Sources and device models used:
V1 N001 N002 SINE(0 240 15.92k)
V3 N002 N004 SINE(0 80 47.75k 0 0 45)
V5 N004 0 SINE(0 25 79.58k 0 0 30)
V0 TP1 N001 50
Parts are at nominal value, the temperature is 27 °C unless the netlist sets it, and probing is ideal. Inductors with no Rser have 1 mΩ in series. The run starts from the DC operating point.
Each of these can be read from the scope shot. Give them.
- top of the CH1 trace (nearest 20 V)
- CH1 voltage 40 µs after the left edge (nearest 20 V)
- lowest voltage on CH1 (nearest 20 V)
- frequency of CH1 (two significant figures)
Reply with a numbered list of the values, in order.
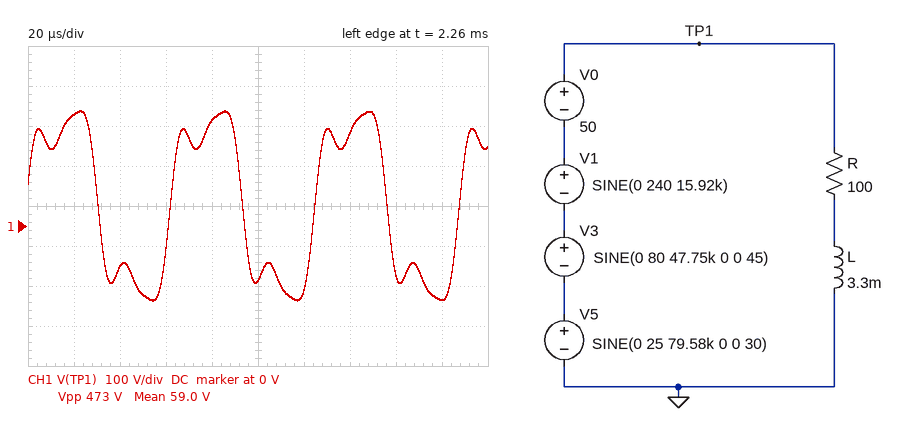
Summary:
1. 280 V
2. -100 V
3. -180 V
4. 16 kHz
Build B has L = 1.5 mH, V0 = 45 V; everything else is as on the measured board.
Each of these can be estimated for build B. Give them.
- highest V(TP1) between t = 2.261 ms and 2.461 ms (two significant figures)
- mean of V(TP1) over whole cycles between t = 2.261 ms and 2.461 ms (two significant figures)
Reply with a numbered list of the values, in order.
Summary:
1. 280 V
2. 45 V
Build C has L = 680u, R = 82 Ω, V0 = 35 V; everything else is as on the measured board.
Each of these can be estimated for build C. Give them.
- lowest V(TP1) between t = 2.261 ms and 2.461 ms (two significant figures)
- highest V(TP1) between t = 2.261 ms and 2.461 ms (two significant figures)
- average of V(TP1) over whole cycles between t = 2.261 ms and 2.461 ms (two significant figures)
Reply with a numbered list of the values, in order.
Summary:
1. -200 V
2. 270 V
3. 35 V
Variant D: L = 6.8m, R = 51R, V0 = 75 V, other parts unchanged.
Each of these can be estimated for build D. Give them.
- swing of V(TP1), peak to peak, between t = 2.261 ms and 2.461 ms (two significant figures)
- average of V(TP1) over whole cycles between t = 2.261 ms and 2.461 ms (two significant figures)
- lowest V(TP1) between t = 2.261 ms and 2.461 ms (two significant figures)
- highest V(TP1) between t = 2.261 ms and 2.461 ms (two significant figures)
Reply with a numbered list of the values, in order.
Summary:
1. 470 V
2. 75 V
3. -160 V
4. 310 V
